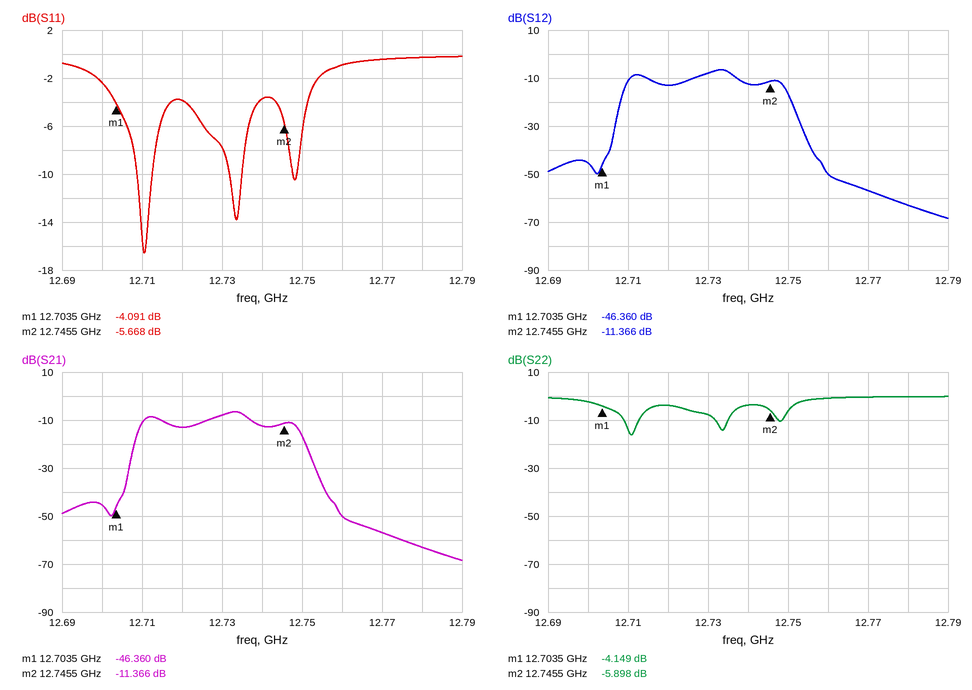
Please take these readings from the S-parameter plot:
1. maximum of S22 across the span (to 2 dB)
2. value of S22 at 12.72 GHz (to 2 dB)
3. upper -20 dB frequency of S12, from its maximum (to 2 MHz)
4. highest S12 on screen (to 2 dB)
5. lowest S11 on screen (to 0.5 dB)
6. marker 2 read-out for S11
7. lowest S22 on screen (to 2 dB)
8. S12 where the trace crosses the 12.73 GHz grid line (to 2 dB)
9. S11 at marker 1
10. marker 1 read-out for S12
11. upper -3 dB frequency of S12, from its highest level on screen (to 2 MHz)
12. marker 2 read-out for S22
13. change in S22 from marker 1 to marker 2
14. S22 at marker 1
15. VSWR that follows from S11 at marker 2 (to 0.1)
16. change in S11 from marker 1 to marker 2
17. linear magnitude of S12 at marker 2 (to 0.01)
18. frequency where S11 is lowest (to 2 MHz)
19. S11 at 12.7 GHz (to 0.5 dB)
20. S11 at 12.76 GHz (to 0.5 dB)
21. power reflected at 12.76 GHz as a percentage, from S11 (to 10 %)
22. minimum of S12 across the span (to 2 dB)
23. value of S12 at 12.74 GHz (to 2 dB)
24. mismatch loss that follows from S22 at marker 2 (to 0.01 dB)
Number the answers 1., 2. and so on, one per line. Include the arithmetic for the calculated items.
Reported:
1. 0 dB
2. -4 dB
3. 12.752 GHz
4. -6 dB
5. -16.5 dB
6. -5.668 dB
7. -16 dB
8. -8 dB
9. -4.091 dB
10. -46.360 dB
11. 12.736 GHz
12. -5.898 dB
13. -5.898 − (-4.149) = -1.749 dB
14. -4.149 dB
15. (1 + 0.5207)/(1 − 0.5207) ≈ 3.2
16. -5.668 − (-4.091) = -1.577 dB
17. 10^(-11.366/20) ≈ 0.27
18. 12.710 GHz
19. -2.5 dB
20. -1.0 dB
21. 10^(-1/10) ≈ 79.4 %, so 80 % to the nearest 10 %
22. -68 dB
23. -12 dB
24. −10 log10(1 − 10^(-5.898/10)) ≈ 1.29 dB
